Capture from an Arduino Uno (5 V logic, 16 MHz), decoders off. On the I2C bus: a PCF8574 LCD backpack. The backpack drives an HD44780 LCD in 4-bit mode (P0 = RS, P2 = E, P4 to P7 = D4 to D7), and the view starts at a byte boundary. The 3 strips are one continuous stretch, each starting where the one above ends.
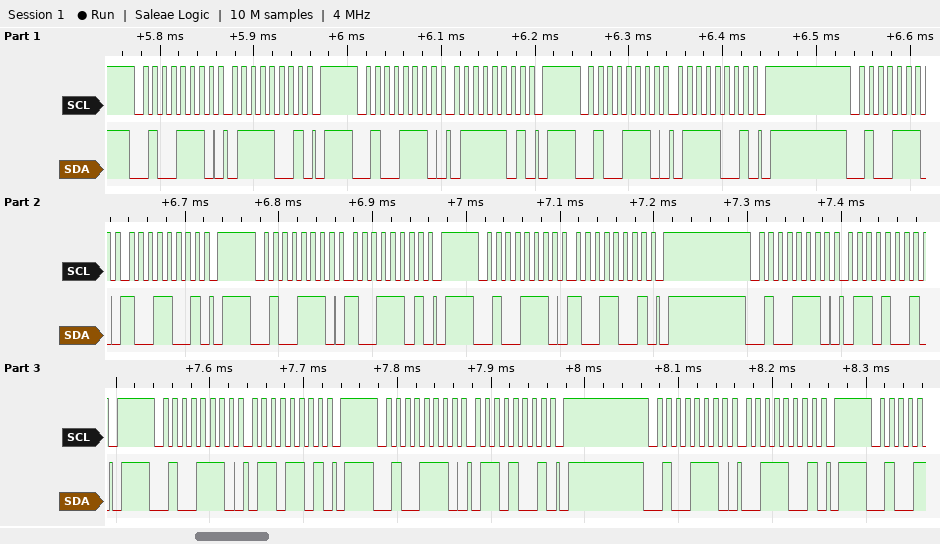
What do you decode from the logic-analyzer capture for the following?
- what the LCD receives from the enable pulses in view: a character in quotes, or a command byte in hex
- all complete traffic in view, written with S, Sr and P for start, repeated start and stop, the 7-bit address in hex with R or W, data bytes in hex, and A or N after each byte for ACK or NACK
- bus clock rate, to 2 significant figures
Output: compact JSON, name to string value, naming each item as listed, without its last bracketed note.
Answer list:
{"what the LCD receives from the enable pulses in view: a character in quotes, or a command byte in hex": "'y'", "all complete traffic in view, written with S, Sr and P for start, repeated start and stop, the 7-bit address in hex with R or W, data bytes in hex, and A or N after each byte for ACK or NACK": "S 27W A 79 A P S 27W A 7D A P S 27W A 79 A P S 27W A 99 A P S 27W A 9D A P S 27W A 99 A P S 27W A 69 A P S 27W A 6D A P S 27W A 69 A P S 27W A 39 A P", "bus clock rate, to 2 significant figures": "100 kHz"}
